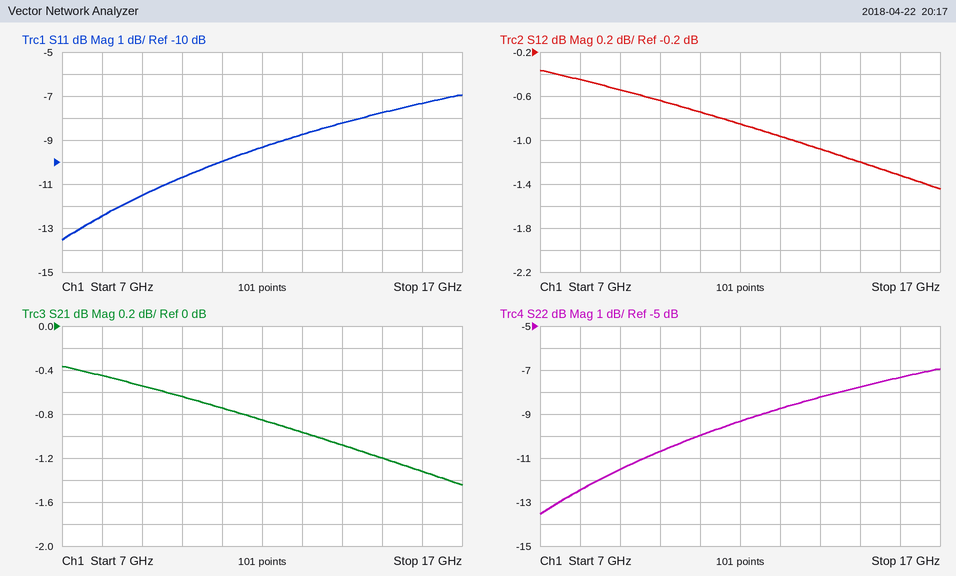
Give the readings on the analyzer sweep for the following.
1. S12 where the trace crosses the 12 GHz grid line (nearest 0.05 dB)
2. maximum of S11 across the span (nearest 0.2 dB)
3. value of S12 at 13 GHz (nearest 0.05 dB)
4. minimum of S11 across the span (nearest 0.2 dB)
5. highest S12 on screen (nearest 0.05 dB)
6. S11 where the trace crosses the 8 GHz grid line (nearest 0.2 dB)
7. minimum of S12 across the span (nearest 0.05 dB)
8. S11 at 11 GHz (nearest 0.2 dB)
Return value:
-0.85 dB
-7.0 dB
-0.95 dB
-13.6 dB
-0.35 dB
-12.4 dB
-1.45 dB
-10.0 dB
